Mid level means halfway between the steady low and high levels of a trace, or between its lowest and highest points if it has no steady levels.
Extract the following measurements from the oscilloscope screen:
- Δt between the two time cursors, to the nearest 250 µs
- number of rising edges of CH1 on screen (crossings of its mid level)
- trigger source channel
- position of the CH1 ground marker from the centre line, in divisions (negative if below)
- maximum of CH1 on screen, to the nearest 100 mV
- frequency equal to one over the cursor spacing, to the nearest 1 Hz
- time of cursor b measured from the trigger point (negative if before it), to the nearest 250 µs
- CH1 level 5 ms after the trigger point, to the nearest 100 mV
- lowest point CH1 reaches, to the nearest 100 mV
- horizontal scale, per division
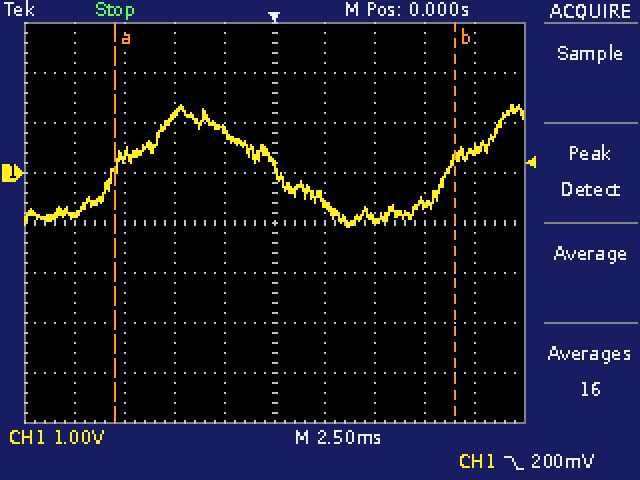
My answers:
17.00 ms
2
CH1
+1.0 div
1.4 V
59 Hz
+9.00 ms
-900 mV
-1.1 V
2.5 ms
